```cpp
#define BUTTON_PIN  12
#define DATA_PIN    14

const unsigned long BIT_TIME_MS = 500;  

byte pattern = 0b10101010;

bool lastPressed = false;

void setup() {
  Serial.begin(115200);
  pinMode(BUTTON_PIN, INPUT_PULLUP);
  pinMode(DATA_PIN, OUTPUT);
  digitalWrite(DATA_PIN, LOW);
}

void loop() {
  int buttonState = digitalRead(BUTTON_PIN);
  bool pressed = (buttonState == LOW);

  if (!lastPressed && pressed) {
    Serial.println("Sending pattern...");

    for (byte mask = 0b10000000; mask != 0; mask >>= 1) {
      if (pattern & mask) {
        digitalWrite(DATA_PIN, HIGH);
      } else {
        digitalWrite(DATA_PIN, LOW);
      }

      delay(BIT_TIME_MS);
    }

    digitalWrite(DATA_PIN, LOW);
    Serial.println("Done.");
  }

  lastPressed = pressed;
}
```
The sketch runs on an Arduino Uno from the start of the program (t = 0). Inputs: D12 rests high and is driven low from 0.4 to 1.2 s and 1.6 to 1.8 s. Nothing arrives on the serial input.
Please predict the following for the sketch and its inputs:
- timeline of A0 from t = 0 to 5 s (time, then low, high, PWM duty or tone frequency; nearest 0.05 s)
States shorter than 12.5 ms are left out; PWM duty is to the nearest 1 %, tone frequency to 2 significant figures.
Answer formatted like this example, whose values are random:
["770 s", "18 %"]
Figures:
["0 s low; 0.4 s high; 0.9 s low; 1.4 s high; 1.9 s low; 2.4 s high; 2.9 s low; 3.4 s high; 3.9 s low"]
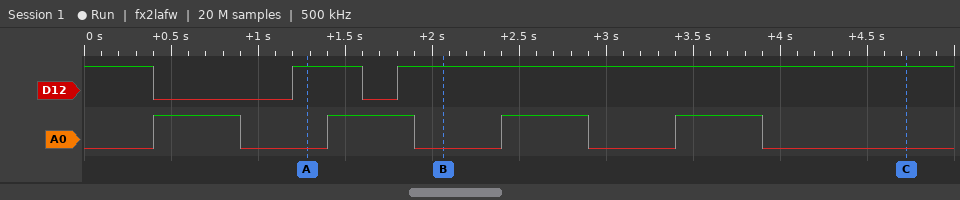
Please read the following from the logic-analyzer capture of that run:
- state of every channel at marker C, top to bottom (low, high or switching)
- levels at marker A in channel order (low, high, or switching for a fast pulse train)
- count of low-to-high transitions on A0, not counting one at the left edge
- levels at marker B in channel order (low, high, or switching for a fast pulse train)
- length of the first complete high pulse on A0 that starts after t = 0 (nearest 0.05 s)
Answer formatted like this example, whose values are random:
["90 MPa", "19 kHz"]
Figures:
["D12 high, A0 low", "D12 high, A0 low", "4", "D12 high, A0 low", "0.50 s"]
